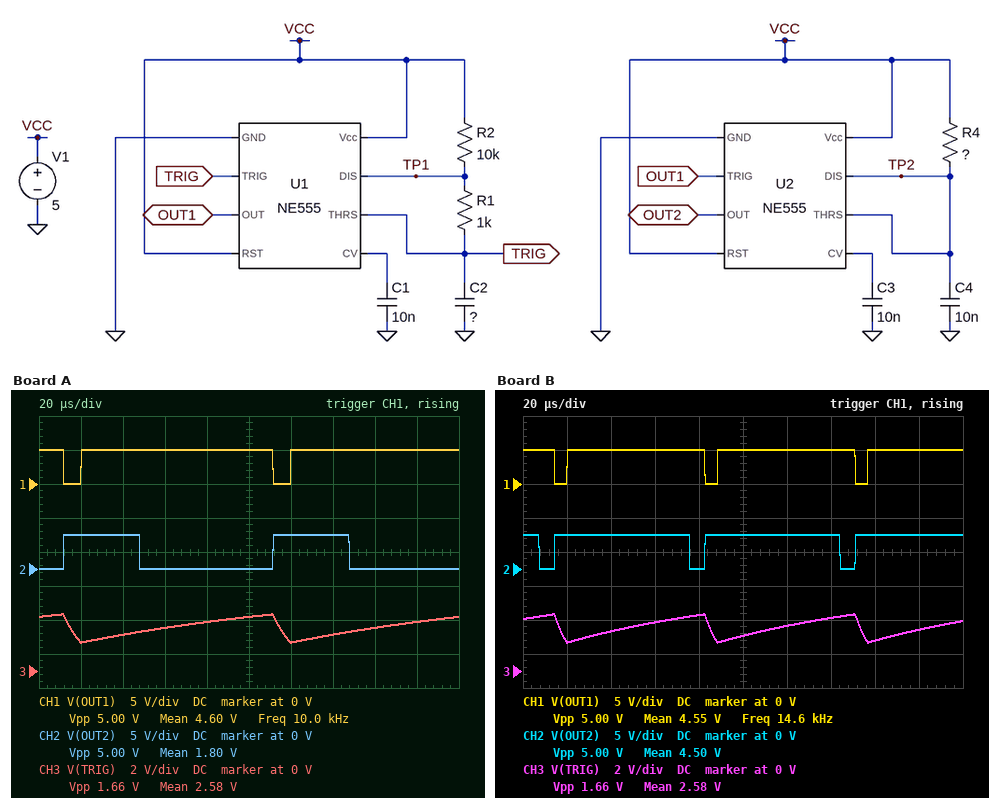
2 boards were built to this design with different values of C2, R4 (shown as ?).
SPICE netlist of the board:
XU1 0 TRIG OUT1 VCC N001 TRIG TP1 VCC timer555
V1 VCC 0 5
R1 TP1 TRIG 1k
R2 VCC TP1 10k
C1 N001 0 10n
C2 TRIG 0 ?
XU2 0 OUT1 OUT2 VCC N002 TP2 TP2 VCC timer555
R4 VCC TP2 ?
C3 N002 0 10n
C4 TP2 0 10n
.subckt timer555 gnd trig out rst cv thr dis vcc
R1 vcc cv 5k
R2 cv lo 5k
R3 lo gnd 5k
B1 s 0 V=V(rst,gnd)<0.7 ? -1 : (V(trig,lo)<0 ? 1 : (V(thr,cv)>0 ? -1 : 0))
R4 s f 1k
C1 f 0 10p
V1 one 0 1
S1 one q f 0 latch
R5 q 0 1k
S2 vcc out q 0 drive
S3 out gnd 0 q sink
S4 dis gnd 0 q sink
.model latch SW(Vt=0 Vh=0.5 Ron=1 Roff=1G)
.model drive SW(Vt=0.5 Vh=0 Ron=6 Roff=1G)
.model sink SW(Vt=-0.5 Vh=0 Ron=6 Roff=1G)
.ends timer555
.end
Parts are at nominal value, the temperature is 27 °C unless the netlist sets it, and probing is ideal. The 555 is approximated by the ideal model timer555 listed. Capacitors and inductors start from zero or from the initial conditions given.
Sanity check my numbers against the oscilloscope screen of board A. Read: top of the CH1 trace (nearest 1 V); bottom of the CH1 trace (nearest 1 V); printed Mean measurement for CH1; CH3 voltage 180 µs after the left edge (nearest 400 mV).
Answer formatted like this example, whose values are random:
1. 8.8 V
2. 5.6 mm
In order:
1. 5 V
2. 0 V
3. 4.60 V
4. 2.8 V
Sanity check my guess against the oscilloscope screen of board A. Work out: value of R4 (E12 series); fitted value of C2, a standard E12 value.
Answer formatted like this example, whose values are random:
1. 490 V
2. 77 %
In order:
1. 3.3 kΩ
2. 12 nF
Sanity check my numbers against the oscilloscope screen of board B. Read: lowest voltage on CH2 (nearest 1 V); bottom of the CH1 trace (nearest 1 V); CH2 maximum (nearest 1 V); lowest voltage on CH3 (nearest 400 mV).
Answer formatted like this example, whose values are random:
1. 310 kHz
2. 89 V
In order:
1. 0 V
2. 0 V
3. 5 V
4. 1.6 V
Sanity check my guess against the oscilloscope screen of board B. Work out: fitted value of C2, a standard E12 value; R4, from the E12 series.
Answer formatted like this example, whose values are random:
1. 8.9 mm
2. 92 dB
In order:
1. 8.2 nF
2. 5.6 kΩ
